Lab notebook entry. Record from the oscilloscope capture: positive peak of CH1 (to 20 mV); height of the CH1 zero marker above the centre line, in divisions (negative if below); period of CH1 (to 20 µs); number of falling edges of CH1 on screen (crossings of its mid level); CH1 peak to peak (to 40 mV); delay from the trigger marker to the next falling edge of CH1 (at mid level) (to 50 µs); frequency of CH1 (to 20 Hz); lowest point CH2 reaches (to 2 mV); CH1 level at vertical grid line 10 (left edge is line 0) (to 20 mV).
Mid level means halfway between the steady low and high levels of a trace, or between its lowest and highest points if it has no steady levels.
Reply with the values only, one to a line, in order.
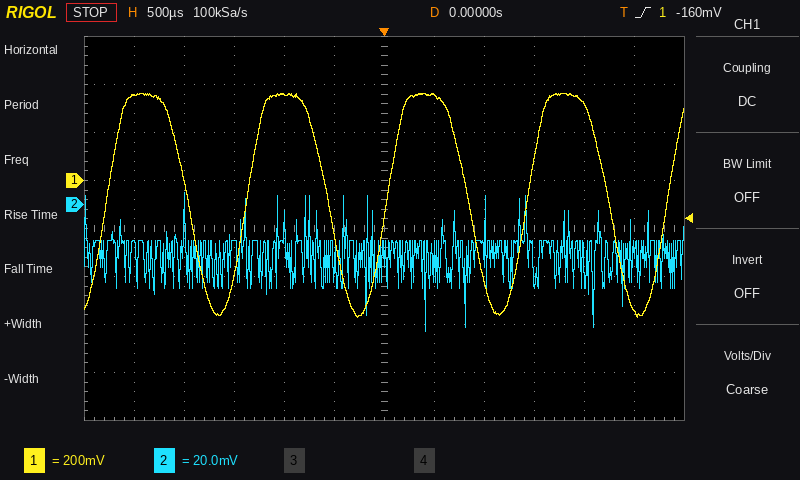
360 mV
+1.0 div
1.40 ms
4
920 mV
850 µs
720 Hz
-52 mV
320 mV
